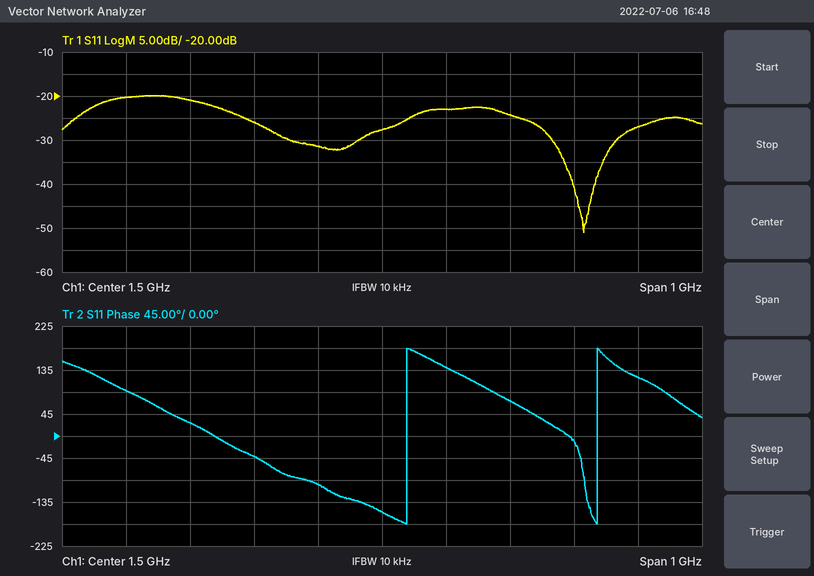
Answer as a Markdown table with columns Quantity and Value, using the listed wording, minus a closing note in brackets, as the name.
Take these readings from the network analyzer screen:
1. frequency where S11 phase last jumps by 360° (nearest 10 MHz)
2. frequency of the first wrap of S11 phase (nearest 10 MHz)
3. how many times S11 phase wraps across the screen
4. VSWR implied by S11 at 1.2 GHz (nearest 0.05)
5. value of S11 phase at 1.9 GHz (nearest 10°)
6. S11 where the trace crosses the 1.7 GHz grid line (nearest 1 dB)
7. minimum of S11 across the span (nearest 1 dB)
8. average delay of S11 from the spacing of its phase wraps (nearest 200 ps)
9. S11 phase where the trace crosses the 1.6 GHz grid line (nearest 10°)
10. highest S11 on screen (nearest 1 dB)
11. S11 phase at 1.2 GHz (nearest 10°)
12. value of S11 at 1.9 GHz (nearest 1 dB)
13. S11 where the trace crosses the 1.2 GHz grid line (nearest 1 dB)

| Quantity | Value |
|---|---|
| frequency where S11 phase last jumps by 360° | 1.84 GHz |
| frequency of the first wrap of S11 phase | 1.54 GHz |
| how many times S11 phase wraps across the screen | 2 |
| VSWR implied by S11 at 1.2 GHz | 1.20 |
| value of S11 phase at 1.9 GHz | 120° |
| S11 where the trace crosses the 1.7 GHz grid line | -24 dB |
| minimum of S11 across the span | -51 dB |
| average delay of S11 from the spacing of its phase wraps | 3.4 ns |
| S11 phase where the trace crosses the 1.6 GHz grid line | 140° |
| highest S11 on screen | -20 dB |
| S11 phase at 1.2 GHz | 30° |
| value of S11 at 1.9 GHz | -27 dB |
| S11 where the trace crosses the 1.2 GHz grid line | -21 dB |
